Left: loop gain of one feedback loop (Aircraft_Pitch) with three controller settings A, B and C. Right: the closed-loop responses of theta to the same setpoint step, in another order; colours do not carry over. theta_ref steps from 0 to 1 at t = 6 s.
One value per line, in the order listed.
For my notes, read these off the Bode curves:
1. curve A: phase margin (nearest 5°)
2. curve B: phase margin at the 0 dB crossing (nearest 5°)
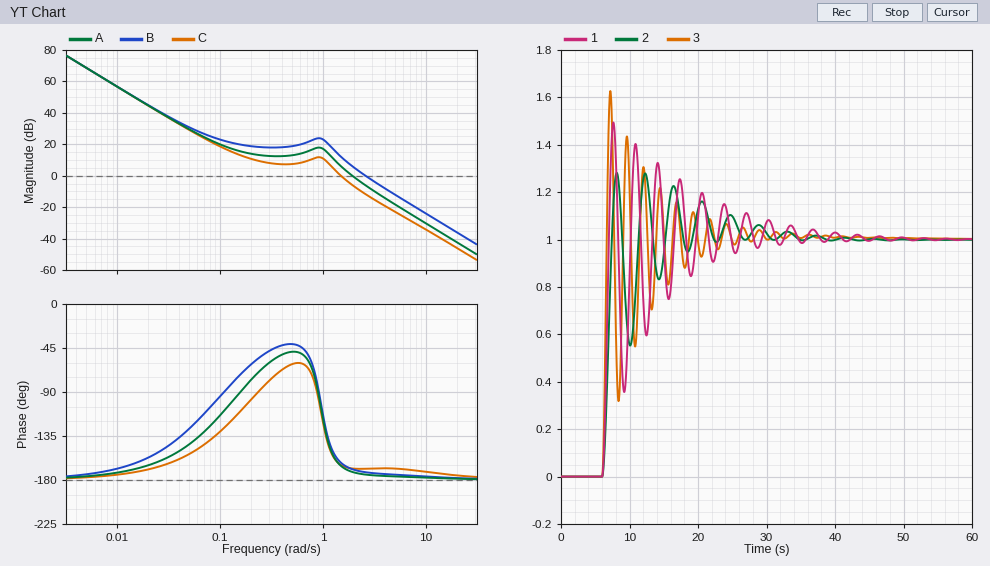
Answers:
10°
10°
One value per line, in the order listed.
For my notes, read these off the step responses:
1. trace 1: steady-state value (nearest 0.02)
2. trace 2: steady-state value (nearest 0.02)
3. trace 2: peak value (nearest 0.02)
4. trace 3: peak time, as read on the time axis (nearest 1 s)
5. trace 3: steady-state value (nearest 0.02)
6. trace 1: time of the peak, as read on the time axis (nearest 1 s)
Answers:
1.00
1.00
1.28
7 s
1.00
8 s
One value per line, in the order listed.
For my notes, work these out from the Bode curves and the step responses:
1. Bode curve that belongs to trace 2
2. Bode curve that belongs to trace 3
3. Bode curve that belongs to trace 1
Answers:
C
B
A
